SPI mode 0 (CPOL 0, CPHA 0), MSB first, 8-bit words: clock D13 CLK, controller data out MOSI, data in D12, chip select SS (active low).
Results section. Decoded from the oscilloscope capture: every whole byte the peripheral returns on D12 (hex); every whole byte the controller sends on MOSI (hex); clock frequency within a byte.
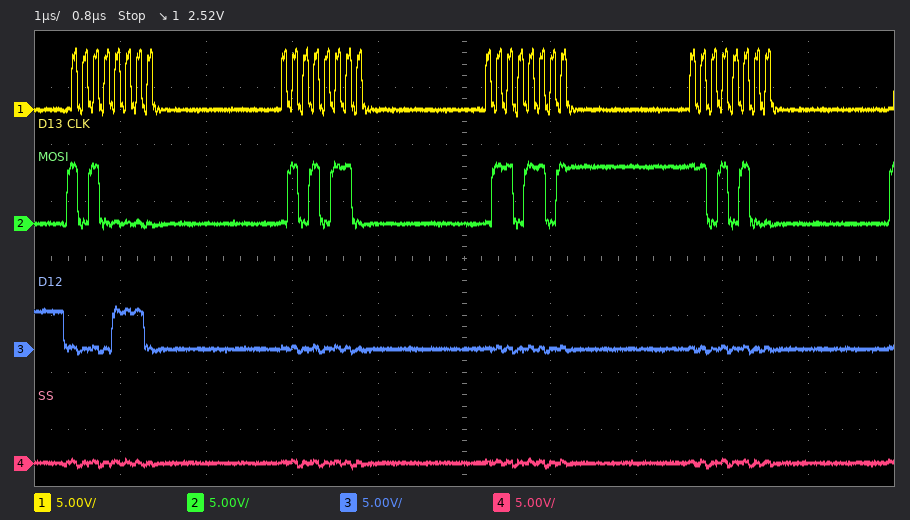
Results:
0E 00 00 00
A0 56 6D D4
8 MHz
